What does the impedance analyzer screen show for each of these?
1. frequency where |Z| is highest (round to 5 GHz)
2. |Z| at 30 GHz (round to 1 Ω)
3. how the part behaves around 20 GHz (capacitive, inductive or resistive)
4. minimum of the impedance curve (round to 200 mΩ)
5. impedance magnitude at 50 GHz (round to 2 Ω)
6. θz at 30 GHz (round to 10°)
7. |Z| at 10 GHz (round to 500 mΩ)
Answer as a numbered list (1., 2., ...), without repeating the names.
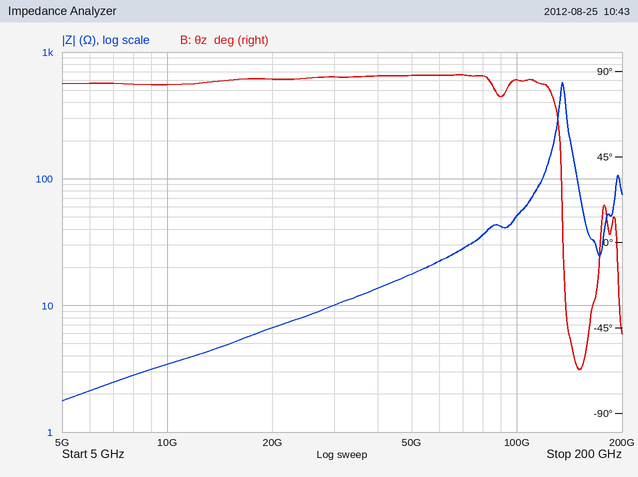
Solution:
1. 135 GHz
2. 10 Ω
3. inductive
4. 1.8 Ω
5. 18 Ω
6. 90°
7. 3.5 Ω
